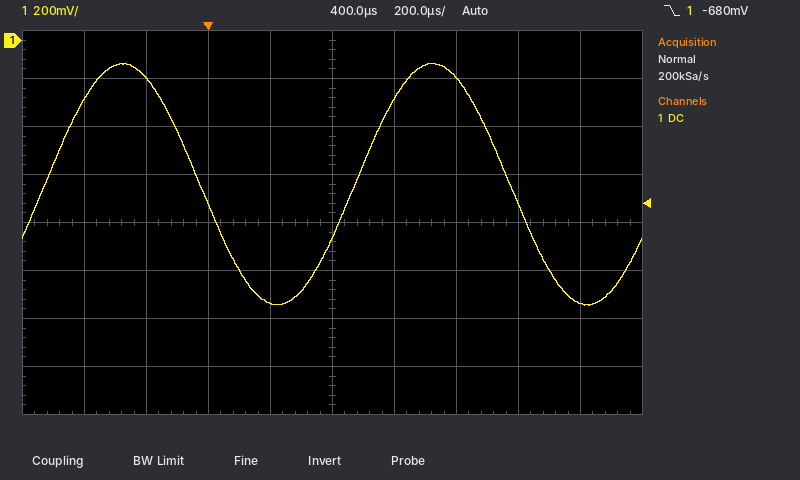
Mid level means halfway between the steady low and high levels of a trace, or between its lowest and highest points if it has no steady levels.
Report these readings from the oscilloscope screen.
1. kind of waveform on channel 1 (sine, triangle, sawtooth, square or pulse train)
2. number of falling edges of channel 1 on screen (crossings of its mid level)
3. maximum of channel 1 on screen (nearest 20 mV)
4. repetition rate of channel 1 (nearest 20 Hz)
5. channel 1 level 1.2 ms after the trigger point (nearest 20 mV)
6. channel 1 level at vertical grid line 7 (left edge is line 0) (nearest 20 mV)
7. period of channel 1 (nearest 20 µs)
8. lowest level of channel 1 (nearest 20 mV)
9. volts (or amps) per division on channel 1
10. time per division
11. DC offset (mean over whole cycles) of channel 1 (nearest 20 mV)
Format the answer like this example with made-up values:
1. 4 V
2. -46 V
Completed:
1. sine
2. 2
3. -100 mV
4. 1.00 kHz
5. -1.10 V
6. -160 mV
7. 1.00 ms
8. -1.10 V
9. 200 mV
10. 200 µs
11. -600 mV
